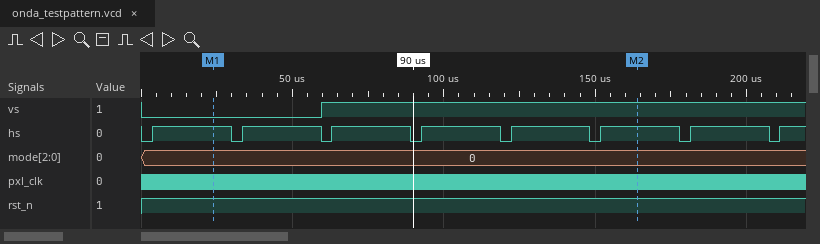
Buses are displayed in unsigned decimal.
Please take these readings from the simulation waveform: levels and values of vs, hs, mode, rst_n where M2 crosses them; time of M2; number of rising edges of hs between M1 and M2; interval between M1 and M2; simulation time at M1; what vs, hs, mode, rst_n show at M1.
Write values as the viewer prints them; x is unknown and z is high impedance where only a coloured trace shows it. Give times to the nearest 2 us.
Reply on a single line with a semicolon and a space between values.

vs=1, hs=1, mode=0, rst_n=1; 164 us; 5; 140 us; 24 us; vs=0, hs=1, mode=0, rst_n=1
